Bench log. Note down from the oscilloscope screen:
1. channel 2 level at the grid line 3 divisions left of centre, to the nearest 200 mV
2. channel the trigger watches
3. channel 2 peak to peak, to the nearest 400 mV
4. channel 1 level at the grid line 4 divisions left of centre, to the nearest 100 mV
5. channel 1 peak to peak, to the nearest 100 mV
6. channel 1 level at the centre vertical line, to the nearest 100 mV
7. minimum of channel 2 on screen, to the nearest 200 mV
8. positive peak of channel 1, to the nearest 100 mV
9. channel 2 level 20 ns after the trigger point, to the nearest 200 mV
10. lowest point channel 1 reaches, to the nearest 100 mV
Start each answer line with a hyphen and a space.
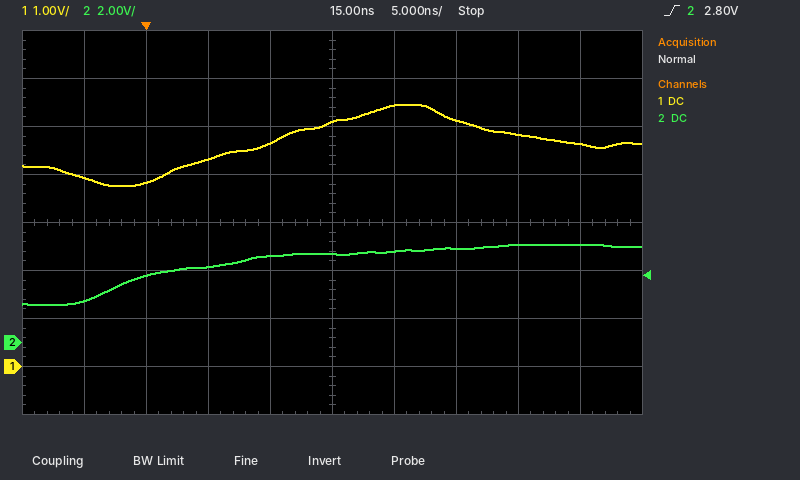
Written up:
- 2.8 V
- channel 2
- 2.4 V
- 3.9 V
- 1.7 V
- 5.1 V
- 1.6 V
- 5.5 V
- 3.8 V
- 3.8 V
